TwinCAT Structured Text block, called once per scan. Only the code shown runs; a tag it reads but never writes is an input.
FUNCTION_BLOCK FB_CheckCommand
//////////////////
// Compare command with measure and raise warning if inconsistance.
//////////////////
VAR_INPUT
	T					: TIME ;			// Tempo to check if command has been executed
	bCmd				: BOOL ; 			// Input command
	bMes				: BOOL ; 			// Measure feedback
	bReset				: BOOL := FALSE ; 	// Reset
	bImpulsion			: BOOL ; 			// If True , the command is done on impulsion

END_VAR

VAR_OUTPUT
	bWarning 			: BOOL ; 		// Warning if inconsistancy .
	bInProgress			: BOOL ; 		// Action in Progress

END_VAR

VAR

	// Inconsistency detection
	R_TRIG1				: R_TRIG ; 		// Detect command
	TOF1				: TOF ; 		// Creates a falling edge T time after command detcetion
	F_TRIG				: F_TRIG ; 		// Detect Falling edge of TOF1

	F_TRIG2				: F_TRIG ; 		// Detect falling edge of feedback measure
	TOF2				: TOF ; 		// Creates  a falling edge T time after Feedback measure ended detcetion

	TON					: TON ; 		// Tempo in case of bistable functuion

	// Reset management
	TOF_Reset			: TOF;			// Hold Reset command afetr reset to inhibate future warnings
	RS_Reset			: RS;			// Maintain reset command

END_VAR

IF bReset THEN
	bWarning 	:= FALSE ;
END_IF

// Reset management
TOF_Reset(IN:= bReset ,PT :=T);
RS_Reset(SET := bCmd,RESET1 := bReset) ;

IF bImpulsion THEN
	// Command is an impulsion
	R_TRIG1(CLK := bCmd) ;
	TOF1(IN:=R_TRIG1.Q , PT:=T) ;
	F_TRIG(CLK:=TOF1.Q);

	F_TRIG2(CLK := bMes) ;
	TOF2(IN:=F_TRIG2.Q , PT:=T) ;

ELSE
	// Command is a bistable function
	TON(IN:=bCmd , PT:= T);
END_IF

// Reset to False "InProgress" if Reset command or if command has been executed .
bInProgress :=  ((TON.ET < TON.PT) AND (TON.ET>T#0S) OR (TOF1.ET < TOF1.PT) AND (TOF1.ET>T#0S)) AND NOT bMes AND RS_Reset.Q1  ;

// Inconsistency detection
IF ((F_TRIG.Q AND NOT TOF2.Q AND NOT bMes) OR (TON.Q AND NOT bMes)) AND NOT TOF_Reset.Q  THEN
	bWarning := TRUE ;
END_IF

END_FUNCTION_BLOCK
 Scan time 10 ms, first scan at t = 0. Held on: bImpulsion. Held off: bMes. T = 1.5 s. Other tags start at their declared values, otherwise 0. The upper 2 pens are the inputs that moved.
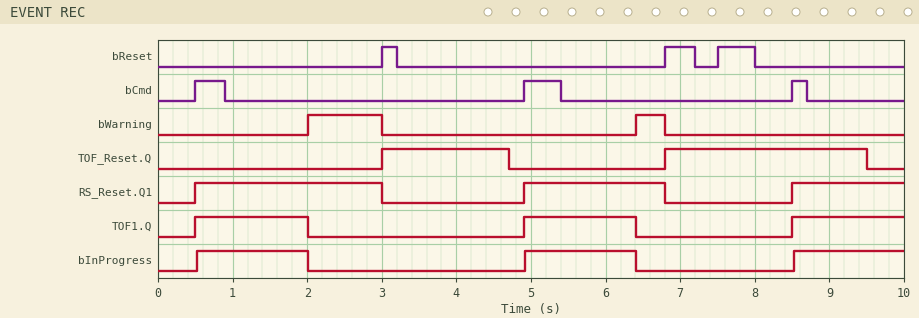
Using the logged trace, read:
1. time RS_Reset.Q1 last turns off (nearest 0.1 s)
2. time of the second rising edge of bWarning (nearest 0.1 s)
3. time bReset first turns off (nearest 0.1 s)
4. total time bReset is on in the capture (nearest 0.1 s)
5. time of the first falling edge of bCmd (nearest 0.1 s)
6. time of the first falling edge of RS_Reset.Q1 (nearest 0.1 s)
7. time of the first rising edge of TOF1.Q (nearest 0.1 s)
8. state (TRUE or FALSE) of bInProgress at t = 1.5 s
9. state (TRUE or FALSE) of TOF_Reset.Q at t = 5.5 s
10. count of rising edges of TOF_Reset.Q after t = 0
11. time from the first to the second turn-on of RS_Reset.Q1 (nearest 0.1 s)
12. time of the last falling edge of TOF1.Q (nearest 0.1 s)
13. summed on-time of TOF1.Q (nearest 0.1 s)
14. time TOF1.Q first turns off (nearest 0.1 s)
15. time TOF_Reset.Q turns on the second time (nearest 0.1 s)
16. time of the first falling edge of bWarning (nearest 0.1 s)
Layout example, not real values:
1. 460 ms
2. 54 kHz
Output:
1. 6.8 s
2. 6.4 s
3. 3.2 s
4. 1.1 s
5. 0.9 s
6. 3.0 s
7. 0.5 s
8. TRUE
9. FALSE
10. 2
11. 4.4 s
12. 6.4 s
13. 4.5 s
14. 2.0 s
15. 6.8 s
16. 3.0 s
